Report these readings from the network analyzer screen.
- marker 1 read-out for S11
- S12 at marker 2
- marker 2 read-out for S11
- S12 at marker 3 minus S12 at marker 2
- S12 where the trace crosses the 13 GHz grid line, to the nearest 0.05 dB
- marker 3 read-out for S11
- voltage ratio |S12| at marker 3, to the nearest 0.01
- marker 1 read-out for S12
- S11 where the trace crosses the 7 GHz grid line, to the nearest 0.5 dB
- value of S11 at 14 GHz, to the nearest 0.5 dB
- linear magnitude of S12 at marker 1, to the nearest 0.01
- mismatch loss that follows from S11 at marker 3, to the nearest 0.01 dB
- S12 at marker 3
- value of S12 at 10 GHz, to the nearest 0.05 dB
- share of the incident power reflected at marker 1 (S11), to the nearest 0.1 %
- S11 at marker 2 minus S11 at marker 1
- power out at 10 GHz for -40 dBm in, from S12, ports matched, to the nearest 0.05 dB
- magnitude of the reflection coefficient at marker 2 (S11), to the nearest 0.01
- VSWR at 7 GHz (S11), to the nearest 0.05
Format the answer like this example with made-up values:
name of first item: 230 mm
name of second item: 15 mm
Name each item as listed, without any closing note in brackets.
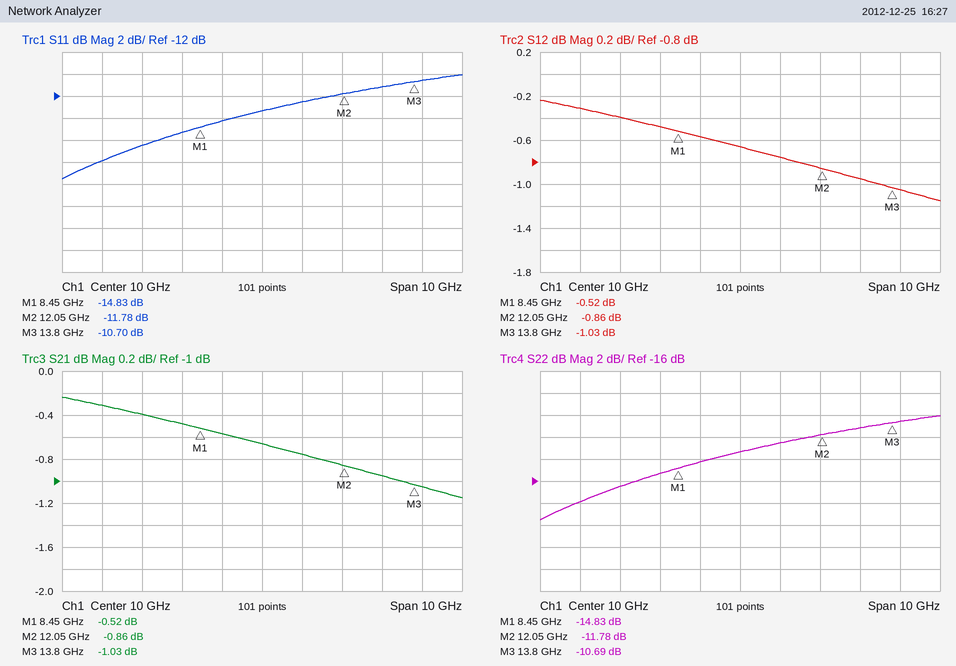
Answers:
marker 1 read-out for S11: -14.83 dB
S12 at marker 2: -0.86 dB
marker 2 read-out for S11: -11.78 dB
S12 at marker 3 minus S12 at marker 2: -0.17 dB
S12 where the trace crosses the 13 GHz grid line, to the nearest 0.05 dB: -0.95 dB
marker 3 read-out for S11: -10.70 dB
voltage ratio |S12| at marker 3, to the nearest 0.01: 0.89
marker 1 read-out for S12: -0.52 dB
S11 where the trace crosses the 7 GHz grid line, to the nearest 0.5 dB: -16.5 dB
value of S11 at 14 GHz, to the nearest 0.5 dB: -10.5 dB
linear magnitude of S12 at marker 1, to the nearest 0.01: 0.94
mismatch loss that follows from S11 at marker 3, to the nearest 0.01 dB: 0.39 dB
S12 at marker 3: -1.03 dB
value of S12 at 10 GHz, to the nearest 0.05 dB: -0.65 dB
share of the incident power reflected at marker 1 (S11), to the nearest 0.1 %: 3.3 %
S11 at marker 2 minus S11 at marker 1: 3.05 dB
power out at 10 GHz for -40 dBm in, from S12, ports matched, to the nearest 0.05 dB: -40.65 dBm
magnitude of the reflection coefficient at marker 2 (S11), to the nearest 0.01: 0.26
VSWR at 7 GHz (S11), to the nearest 0.05: 1.35
